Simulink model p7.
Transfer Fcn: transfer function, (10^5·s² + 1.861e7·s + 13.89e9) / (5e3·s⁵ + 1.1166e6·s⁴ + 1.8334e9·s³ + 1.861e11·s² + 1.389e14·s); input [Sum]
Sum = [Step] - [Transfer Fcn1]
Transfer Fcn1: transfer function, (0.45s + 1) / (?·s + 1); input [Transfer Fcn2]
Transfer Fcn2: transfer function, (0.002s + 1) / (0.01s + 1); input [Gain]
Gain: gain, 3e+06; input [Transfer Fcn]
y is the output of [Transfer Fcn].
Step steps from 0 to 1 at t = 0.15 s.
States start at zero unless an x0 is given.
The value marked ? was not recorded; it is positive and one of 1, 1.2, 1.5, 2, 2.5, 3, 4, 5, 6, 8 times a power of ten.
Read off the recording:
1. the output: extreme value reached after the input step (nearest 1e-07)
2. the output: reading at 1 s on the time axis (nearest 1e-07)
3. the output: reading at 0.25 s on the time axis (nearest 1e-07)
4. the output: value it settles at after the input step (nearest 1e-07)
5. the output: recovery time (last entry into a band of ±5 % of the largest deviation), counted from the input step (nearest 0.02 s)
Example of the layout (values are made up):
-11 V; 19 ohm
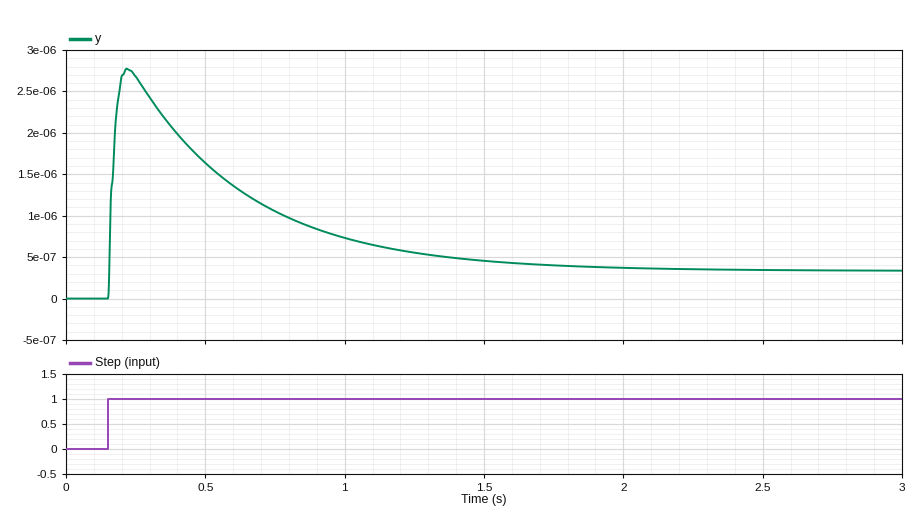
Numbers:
0.0000028; 0.0000007; 0.0000027; 0.0000003; 1.30 s
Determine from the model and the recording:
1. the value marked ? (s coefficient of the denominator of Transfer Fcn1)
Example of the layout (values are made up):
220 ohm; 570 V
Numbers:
4
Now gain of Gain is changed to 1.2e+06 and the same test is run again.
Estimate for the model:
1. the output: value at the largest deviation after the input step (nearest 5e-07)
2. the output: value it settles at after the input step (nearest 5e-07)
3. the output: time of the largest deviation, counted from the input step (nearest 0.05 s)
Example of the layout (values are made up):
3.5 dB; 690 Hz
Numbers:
0.0000060; 0.0000010; 0.15 s
